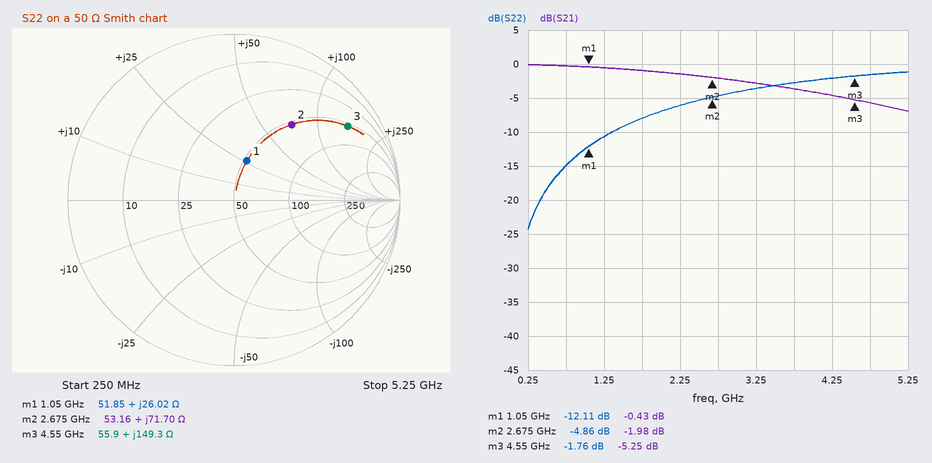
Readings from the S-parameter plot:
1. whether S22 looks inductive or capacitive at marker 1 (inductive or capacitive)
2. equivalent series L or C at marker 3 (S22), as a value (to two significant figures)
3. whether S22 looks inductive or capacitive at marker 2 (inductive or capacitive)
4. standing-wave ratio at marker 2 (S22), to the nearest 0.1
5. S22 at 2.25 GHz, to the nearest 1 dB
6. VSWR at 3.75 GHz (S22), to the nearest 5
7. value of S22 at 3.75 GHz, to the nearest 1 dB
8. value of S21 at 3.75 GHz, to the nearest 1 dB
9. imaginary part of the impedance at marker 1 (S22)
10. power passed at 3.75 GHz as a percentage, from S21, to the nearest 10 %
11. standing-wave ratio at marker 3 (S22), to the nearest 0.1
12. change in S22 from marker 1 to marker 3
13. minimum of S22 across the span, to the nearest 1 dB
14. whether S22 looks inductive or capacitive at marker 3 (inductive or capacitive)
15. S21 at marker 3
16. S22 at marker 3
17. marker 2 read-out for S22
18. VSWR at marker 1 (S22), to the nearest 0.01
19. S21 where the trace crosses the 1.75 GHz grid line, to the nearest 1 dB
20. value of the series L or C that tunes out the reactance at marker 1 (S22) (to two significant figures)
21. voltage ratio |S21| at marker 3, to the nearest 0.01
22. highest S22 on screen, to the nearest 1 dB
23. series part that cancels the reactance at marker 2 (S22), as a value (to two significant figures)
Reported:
inductive
5.2 nH
inductive
3.7
-6 dB
5
-3 dB
-4 dB
+26.02 Ω
40 %
9.9
10.35 dB
-24 dB
inductive
-5.25 dB
-1.76 dB
-4.86 dB
1.66
-1 dB
5.8 pF
0.55
-1 dB
830 fF
